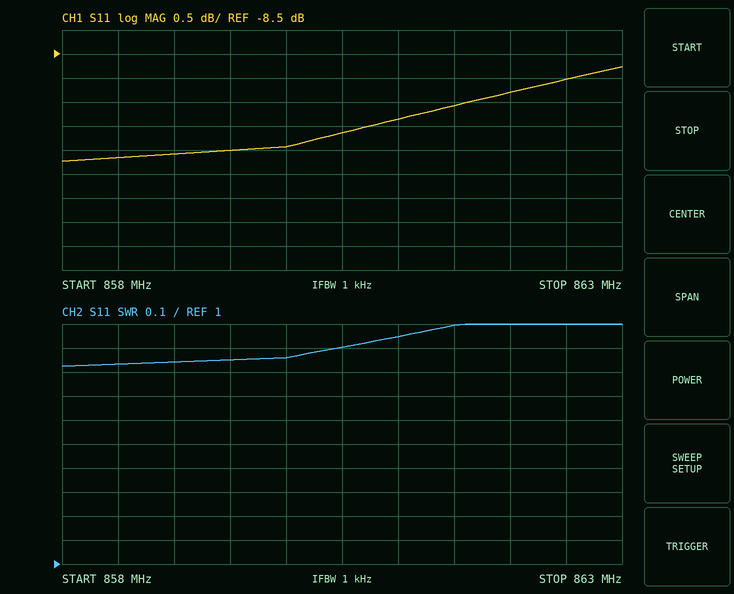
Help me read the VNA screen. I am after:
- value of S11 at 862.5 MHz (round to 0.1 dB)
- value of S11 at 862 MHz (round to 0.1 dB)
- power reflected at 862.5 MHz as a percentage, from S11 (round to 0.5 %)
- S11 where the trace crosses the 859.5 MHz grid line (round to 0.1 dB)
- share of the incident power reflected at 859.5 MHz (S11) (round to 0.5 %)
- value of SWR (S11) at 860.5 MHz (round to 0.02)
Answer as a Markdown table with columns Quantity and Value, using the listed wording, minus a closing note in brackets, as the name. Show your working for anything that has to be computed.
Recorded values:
| Quantity | Value |
|---|---|
| value of S11 at 862.5 MHz | -9.0 dB |
| value of S11 at 862 MHz | -9.3 dB |
| power reflected at 862.5 MHz as a percentage, from S11 | 10^(-9/10) ≈ 12.6 %, so 12.5 % to the nearest 0.5 % |
| S11 where the trace crosses the 859.5 MHz grid line | -10.5 dB |
| share of the incident power reflected at 859.5 MHz (S11) | 10^(-10.5/10) ≈ 8.91 %, so 9.0 % to the nearest 0.5 % |
| value of SWR (S11) at 860.5 MHz | 1.90 |
